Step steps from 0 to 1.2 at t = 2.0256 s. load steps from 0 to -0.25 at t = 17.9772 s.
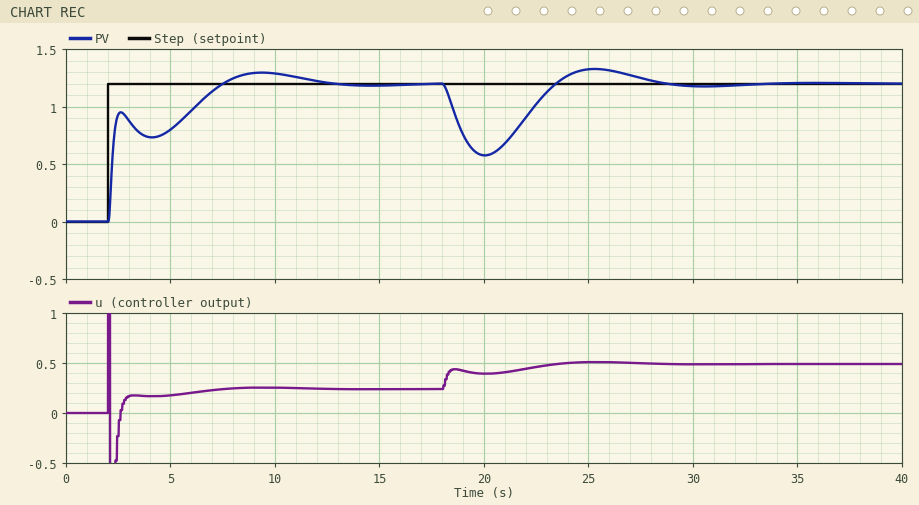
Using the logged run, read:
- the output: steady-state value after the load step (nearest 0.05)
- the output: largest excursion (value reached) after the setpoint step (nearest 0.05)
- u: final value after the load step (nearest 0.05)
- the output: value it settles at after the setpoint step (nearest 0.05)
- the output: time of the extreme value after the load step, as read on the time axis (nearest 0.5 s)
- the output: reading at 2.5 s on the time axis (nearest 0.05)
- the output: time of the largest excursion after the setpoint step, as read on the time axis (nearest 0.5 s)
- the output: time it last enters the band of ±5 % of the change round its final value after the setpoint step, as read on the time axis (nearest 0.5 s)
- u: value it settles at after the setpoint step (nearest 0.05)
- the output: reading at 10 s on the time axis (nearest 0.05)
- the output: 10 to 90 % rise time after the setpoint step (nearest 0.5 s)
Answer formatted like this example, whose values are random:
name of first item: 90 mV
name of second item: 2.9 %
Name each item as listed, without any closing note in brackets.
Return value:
the output: steady-state value after the load step: 1.20
the output: largest excursion (value reached) after the setpoint step: 1.30
u: final value after the load step: 0.50
the output: value it settles at after the setpoint step: 1.20
the output: time of the extreme value after the load step, as read on the time axis: 20.0 s
the output: reading at 2.5 s on the time axis: 0.95
the output: time of the largest excursion after the setpoint step, as read on the time axis: 9.5 s
the output: time it last enters the band of ±5 % of the change round its final value after the setpoint step, as read on the time axis: 11.0 s
u: value it settles at after the setpoint step: 0.25
the output: reading at 10 s on the time axis: 1.30
the output: 10 to 90 % rise time after the setpoint step: 4.5 s
